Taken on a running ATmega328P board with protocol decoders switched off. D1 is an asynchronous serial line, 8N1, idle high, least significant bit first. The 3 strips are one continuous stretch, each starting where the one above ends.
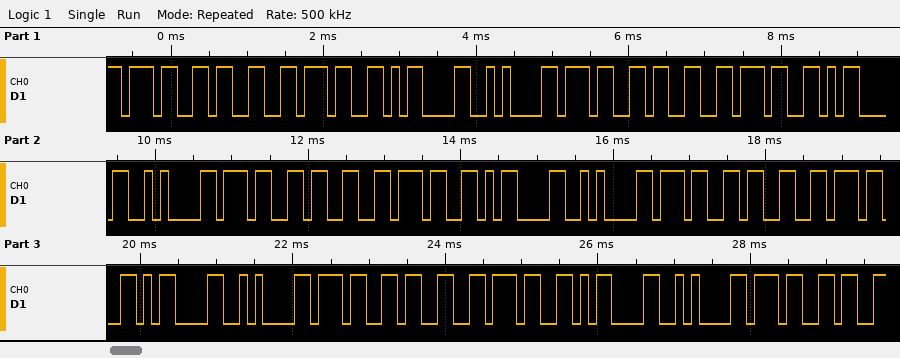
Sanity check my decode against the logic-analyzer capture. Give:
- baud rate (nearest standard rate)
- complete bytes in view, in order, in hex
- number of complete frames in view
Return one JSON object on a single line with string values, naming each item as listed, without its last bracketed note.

{"baud rate": "9600 baud", "complete bytes in view, in order, in hex": "37 33 37 0D 0A 37 33 37 0D 0A 37 33 37 0D 0A 37 33 37 0D 0A 37 33 37 0D 0A 37", "number of complete frames in view": "26"}
